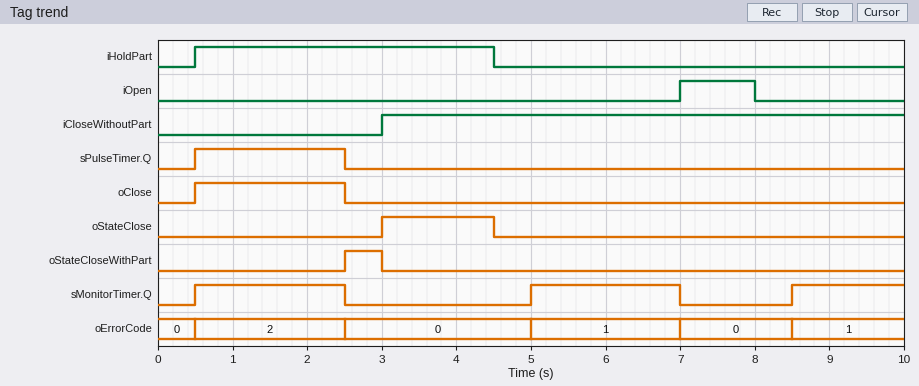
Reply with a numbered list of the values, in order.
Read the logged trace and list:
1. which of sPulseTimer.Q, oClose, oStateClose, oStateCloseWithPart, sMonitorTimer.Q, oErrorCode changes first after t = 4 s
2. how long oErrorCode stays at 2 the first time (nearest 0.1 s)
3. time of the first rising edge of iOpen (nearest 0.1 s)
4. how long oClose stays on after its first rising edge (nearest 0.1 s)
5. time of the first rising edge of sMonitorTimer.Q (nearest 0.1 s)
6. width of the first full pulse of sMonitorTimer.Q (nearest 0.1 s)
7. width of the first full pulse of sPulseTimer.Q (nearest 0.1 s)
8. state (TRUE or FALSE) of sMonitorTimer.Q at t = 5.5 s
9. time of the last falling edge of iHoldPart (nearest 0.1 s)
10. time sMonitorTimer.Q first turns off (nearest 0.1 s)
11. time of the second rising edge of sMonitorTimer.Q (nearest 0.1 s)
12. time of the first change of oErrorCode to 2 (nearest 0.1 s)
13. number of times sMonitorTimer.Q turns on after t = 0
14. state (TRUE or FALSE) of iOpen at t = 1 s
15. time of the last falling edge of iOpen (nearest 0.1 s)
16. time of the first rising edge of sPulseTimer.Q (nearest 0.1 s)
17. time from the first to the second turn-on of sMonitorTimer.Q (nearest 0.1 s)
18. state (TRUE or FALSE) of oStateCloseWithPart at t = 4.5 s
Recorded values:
1. oStateClose
2. 2.0 s
3. 7.0 s
4. 2.0 s
5. 0.5 s
6. 2.0 s
7. 2.0 s
8. TRUE
9. 4.5 s
10. 2.5 s
11. 5.0 s
12. 0.5 s
13. 3
14. FALSE
15. 8.0 s
16. 0.5 s
17. 4.5 s
18. FALSE
